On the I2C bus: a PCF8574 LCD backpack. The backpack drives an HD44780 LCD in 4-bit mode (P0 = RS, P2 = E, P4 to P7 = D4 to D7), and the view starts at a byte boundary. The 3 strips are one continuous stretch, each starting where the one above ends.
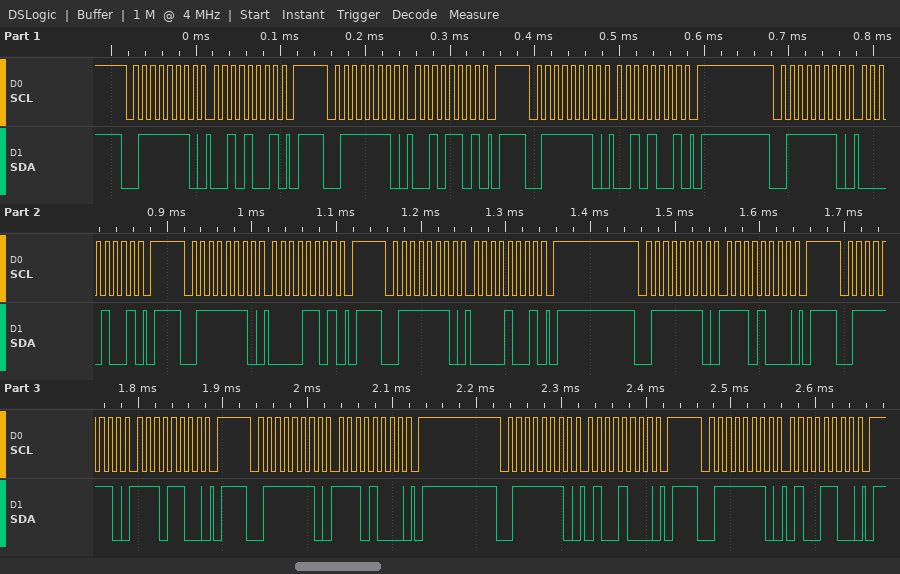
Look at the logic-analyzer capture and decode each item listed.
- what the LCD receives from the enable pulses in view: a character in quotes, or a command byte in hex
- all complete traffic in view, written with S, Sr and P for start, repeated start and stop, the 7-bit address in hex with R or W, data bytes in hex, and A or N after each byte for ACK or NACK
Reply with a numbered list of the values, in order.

1. ' '
2. S 3FW A 29 A P S 3FW A 2D A P S 3FW A 29 A P S 3FW A 09 A P S 3FW A 0D A P S 3FW A 09 A P S 3FW A E8 A P S 3FW A EC A P S 3FW A E8 A P S 3FW A 48 A P S 3FW A 4C A P
